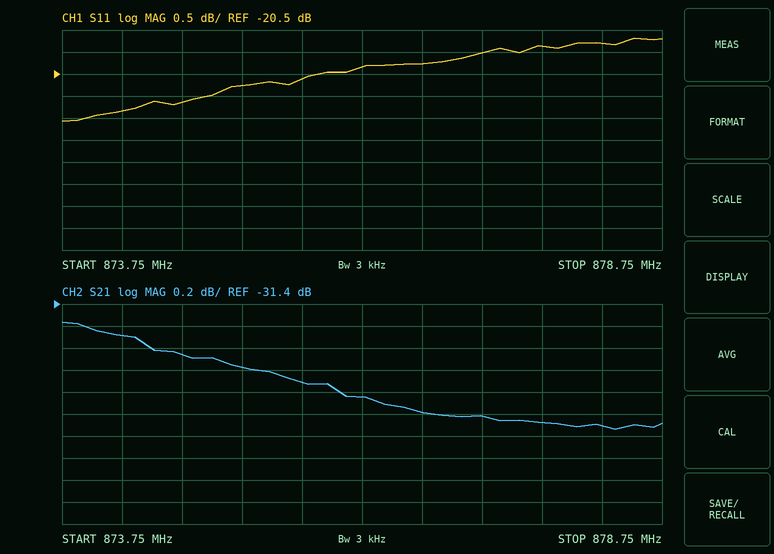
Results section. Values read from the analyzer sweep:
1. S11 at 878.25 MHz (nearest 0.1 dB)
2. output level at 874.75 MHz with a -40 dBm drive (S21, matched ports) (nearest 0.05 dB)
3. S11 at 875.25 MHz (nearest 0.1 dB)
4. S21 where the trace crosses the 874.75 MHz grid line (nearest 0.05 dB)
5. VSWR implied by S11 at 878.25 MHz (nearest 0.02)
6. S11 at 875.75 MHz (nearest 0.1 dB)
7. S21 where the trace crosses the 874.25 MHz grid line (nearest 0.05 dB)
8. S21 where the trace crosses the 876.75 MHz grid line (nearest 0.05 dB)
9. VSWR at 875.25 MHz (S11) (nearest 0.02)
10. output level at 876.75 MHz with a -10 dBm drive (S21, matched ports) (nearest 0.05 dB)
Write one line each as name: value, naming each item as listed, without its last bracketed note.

S11 at 878.25 MHz: -19.8 dB
output level at 874.75 MHz with a -40 dBm drive (S21, matched ports): -71.85 dBm
S11 at 875.25 MHz: -20.8 dB
S21 where the trace crosses the 874.75 MHz grid line: -31.85 dB
VSWR implied by S11 at 878.25 MHz: 1.22
S11 at 875.75 MHz: -20.6 dB
S21 where the trace crosses the 874.25 MHz grid line: -31.70 dB
S21 where the trace crosses the 876.75 MHz grid line: -32.40 dB
VSWR at 875.25 MHz (S11): 1.20
output level at 876.75 MHz with a -10 dBm drive (S21, matched ports): -42.40 dBm
